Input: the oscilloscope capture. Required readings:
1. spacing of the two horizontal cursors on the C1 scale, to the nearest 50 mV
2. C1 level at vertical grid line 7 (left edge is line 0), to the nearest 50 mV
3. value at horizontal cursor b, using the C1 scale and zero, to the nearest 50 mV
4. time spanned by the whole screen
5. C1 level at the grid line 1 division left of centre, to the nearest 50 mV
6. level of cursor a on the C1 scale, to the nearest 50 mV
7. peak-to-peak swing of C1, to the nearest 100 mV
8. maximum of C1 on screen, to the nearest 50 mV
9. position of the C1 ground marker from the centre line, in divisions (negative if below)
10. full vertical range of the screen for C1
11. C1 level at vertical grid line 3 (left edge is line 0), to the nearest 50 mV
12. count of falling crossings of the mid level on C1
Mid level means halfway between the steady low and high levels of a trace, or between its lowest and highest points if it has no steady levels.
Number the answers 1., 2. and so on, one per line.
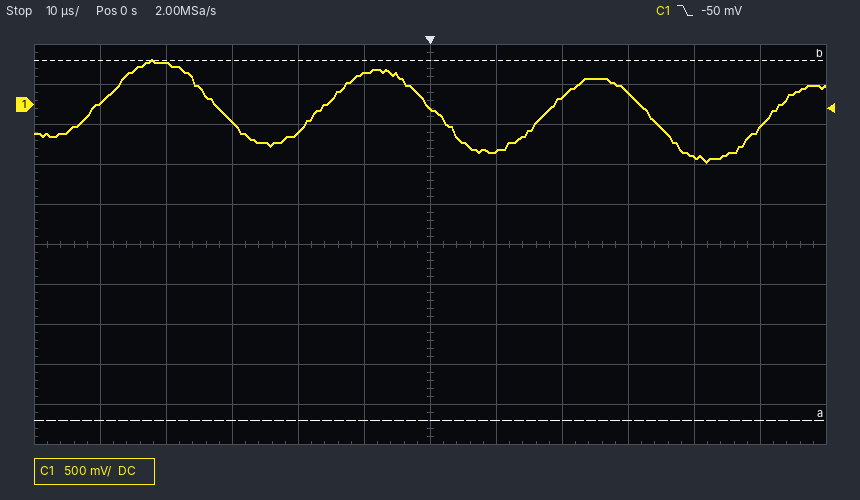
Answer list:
1. 4.50 V
2. -600 mV
3. 550 mV
4. 120 µs
5. 400 mV
6. -3.95 V
7. 1.30 V
8. 550 mV
9. +3.5 div
10. 5 V
11. -200 mV
12. 3
